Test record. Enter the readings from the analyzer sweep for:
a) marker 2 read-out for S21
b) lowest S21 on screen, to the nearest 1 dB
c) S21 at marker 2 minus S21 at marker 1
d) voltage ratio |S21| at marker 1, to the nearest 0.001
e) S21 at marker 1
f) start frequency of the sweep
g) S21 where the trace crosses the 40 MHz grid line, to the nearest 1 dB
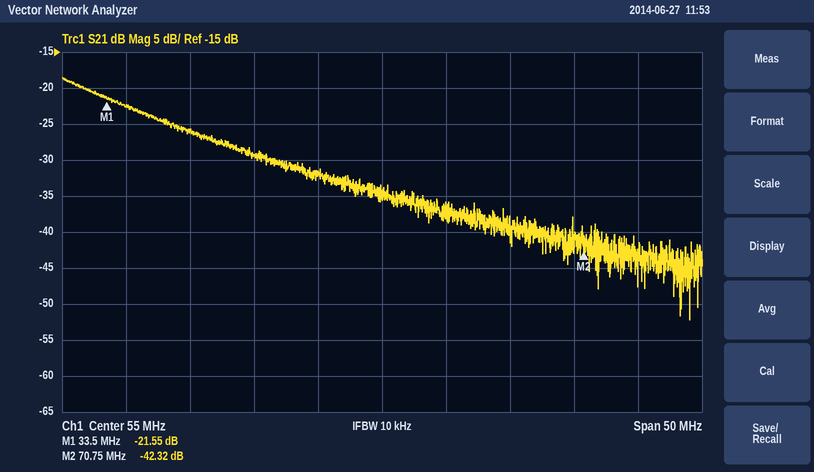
-42.32 dB
-52 dB
-20.77 dB
0.084
-21.55 dB
30 MHz
-26 dB
